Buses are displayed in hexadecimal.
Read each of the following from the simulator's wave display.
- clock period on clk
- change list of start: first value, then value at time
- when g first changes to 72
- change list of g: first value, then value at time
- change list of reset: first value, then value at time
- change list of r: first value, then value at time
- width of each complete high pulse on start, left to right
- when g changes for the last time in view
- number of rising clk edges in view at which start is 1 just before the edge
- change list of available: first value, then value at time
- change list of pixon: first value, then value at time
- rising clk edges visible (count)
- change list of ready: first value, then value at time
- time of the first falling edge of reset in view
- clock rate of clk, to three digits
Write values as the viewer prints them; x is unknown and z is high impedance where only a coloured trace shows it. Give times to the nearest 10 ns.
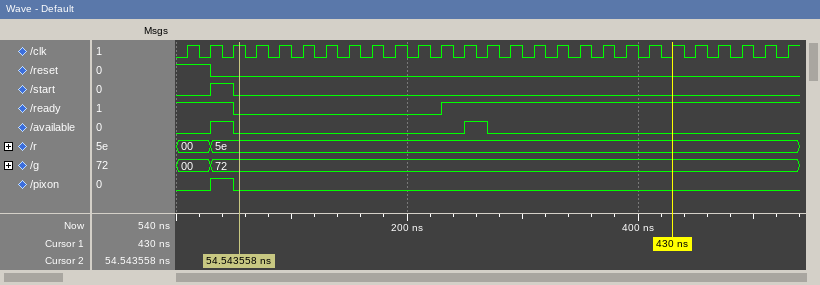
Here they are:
20 ns
0, 1 at 30 ns, 0 at 50 ns
30 ns
00, 72 at 30 ns
1, 0 at 30 ns
00, 5e at 30 ns
20 ns
30 ns
1
0, 1 at 30 ns, 0 at 50 ns, 1 at 250 ns, 0 at 270 ns
0, 1 at 30 ns, 0 at 50 ns
27
1, 0 at 50 ns, 1 at 230 ns
30 ns
50.0 MHz
